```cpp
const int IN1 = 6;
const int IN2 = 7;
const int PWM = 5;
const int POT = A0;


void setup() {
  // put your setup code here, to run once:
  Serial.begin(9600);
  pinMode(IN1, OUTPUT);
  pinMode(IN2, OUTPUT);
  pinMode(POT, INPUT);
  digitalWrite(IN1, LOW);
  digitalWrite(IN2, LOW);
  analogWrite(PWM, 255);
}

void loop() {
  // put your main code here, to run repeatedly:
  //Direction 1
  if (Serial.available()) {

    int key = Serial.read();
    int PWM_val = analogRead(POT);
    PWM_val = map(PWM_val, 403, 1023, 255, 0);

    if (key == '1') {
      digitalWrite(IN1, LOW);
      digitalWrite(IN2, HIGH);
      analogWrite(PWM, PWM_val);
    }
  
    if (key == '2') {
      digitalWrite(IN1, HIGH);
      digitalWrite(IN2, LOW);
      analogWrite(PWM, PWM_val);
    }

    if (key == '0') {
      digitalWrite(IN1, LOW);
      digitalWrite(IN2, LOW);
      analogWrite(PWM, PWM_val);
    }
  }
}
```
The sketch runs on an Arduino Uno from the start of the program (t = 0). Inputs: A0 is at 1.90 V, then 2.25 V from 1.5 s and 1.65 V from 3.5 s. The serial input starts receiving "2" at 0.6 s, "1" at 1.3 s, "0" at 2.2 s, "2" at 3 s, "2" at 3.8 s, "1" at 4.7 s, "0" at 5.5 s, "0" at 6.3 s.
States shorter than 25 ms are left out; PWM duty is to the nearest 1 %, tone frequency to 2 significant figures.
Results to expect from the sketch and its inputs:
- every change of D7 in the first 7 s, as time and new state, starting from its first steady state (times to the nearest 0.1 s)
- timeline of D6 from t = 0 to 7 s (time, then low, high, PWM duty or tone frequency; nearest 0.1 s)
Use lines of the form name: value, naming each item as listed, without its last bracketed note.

every change of D7 in the first 7 s, as time and new state, starting from its first steady state: 0 s low; 1.3 s high; 2.2 s low; 4.7 s high; 5.5 s low
timeline of D6 from t = 0 to 7 s: 0 s low; 0.6 s high; 1.3 s low; 3 s high; 4.7 s low
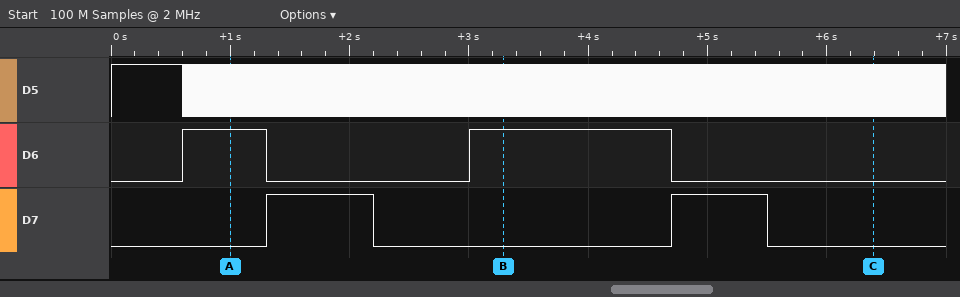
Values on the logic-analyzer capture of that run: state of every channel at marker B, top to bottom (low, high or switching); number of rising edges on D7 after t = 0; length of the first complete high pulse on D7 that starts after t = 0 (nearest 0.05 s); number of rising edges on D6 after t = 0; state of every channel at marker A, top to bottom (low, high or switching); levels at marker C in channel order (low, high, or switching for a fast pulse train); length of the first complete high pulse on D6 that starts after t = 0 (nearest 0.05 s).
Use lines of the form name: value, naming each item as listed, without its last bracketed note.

state of every channel at marker B, top to bottom: D5 switching, D6 high, D7 low
number of rising edges on D7 after t = 0: 2
length of the first complete high pulse on D7 that starts after t = 0: 0.90 s
number of rising edges on D6 after t = 0: 2
state of every channel at marker A, top to bottom: D5 switching, D6 high, D7 low
levels at marker C in channel order: D5 switching, D6 low, D7 low
length of the first complete high pulse on D6 that starts after t = 0: 0.70 s
